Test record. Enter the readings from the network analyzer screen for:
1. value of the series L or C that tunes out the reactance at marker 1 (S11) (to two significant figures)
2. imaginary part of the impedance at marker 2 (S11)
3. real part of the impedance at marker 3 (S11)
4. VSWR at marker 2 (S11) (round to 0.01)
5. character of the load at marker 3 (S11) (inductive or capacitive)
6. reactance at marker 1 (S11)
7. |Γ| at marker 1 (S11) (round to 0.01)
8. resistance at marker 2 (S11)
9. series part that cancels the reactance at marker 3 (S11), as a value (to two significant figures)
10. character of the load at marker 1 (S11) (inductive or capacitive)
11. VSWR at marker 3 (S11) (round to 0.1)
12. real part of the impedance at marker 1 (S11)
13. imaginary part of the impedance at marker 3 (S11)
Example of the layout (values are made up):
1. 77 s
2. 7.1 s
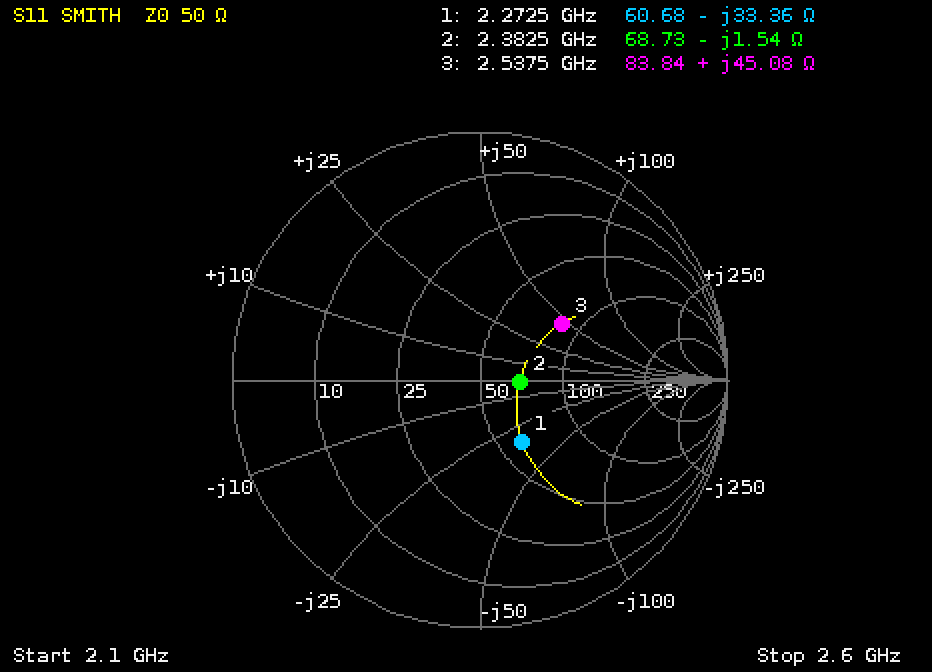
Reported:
1. 2.3 nH
2. -1.54 Ω
3. 83.84 Ω
4. 1.38
5. inductive
6. -33.36 Ω
7. 0.30
8. 68.73 Ω
9. 1.4 pF
10. capacitive
11. 2.3
12. 60.68 Ω
13. +45.08 Ω
